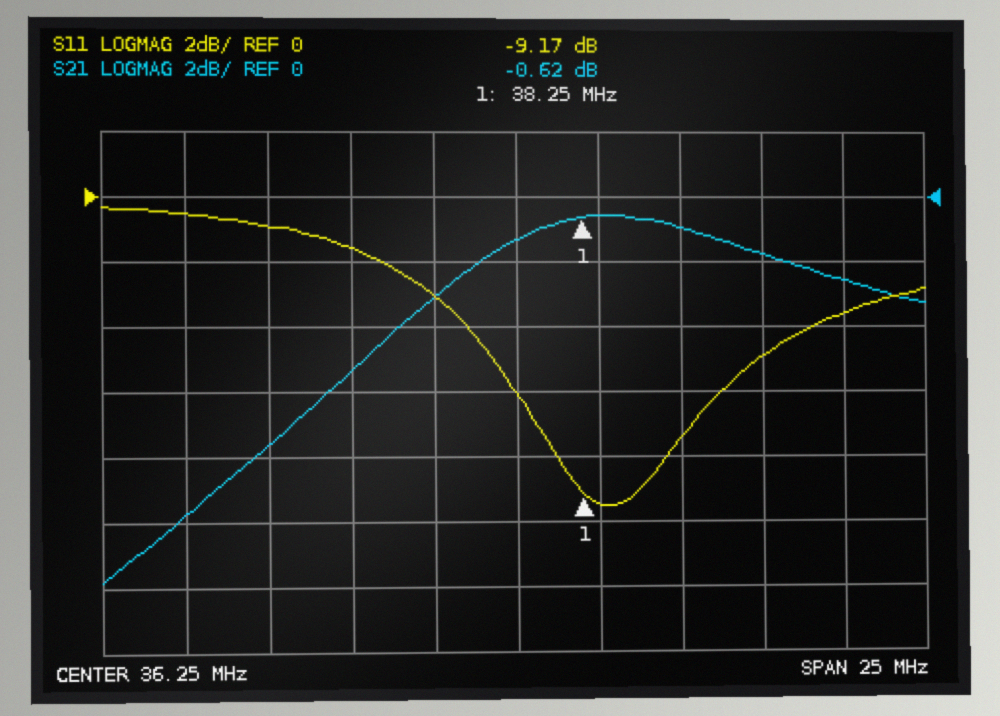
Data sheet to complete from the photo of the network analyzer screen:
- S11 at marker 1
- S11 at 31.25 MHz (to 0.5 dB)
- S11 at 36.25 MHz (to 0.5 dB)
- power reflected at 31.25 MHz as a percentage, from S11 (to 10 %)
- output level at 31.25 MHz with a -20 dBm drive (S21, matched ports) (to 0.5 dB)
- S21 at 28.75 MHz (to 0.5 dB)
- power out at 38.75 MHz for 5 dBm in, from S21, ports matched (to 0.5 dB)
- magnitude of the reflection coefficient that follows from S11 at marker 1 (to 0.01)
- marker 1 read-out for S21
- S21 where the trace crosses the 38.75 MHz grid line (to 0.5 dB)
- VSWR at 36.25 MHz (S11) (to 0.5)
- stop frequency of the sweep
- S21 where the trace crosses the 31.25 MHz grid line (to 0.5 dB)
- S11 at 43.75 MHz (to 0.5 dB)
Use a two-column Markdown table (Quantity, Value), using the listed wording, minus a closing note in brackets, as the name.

| Quantity | Value |
|---|---|
| S11 at marker 1 | -9.17 dB |
| S11 at 31.25 MHz | -1.5 dB |
| S11 at 36.25 MHz | -6.0 dB |
| power reflected at 31.25 MHz as a percentage, from S11 | 70 % |
| output level at 31.25 MHz with a -20 dBm drive (S21, matched ports) | -25.5 dBm |
| S21 at 28.75 MHz | -7.5 dB |
| power out at 38.75 MHz for 5 dBm in, from S21, ports matched | 4.5 dBm |
| magnitude of the reflection coefficient that follows from S11 at marker 1 | 0.35 |
| marker 1 read-out for S21 | -0.62 dB |
| S21 where the trace crosses the 38.75 MHz grid line | -0.5 dB |
| VSWR at 36.25 MHz (S11) | 3.0 |
| stop frequency of the sweep | 48.75 MHz |
| S21 where the trace crosses the 31.25 MHz grid line | -5.5 dB |
| S11 at 43.75 MHz | -5.0 dB |
